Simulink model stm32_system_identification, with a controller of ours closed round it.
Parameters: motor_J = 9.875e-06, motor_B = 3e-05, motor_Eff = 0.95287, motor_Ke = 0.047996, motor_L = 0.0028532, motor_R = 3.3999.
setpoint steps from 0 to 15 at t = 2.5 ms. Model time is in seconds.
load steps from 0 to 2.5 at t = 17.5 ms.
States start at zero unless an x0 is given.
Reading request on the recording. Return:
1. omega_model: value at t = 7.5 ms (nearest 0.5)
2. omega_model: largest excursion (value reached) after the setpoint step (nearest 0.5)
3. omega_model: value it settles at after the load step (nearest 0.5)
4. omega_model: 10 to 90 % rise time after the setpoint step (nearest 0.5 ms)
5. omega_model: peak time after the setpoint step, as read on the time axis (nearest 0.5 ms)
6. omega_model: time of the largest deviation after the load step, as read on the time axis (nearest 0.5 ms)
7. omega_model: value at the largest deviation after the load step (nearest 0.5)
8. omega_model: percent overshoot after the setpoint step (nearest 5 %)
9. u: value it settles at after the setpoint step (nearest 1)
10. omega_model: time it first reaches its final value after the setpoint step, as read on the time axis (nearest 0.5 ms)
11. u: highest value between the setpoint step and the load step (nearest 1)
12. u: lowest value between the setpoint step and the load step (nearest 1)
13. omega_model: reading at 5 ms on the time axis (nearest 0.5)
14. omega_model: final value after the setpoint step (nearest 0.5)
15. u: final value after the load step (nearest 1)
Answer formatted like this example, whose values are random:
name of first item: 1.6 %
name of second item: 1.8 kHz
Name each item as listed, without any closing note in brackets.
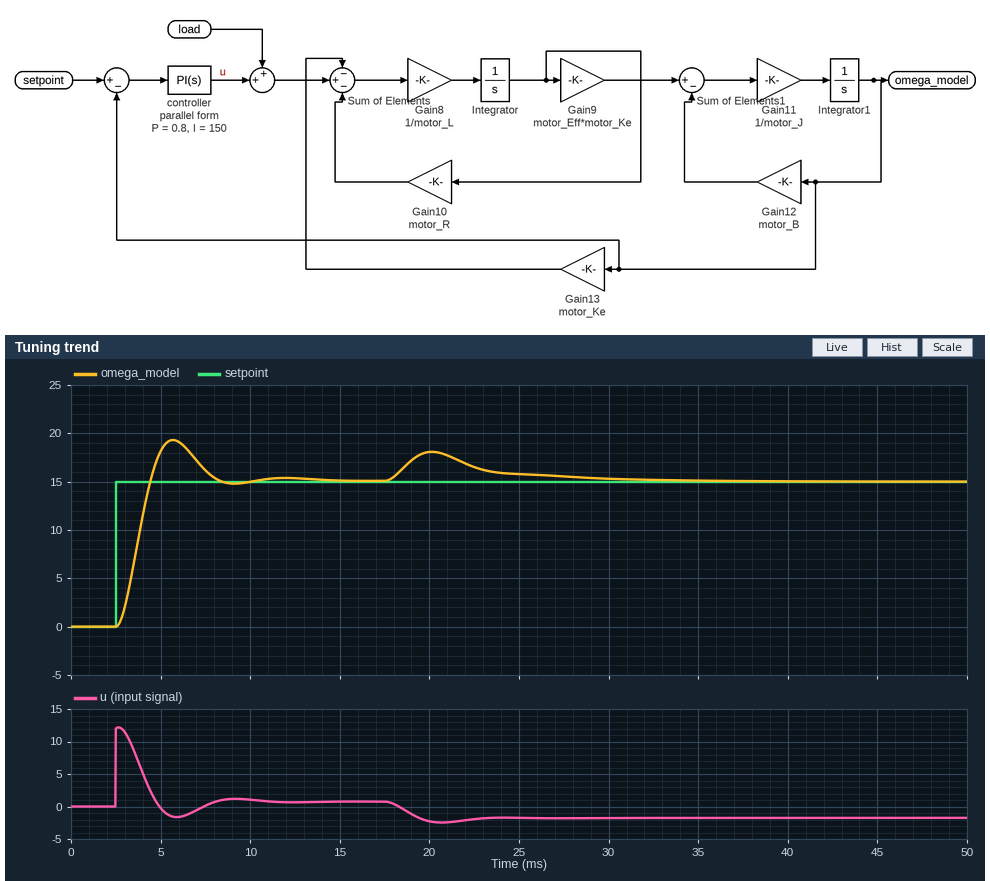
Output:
omega_model: value at t = 7.5 ms: 16.0
omega_model: largest excursion (value reached) after the setpoint step: 19.5
omega_model: value it settles at after the load step: 15.0
omega_model: 10 to 90 % rise time after the setpoint step: 1.5 ms
omega_model: peak time after the setpoint step, as read on the time axis: 5.5 ms
omega_model: time of the largest deviation after the load step, as read on the time axis: 20.0 ms
omega_model: value at the largest deviation after the load step: 18.0
omega_model: percent overshoot after the setpoint step: 30 %
u: value it settles at after the setpoint step: 1
omega_model: time it first reaches its final value after the setpoint step, as read on the time axis: 4.5 ms
u: highest value between the setpoint step and the load step: 12
u: lowest value between the setpoint step and the load step: -2
omega_model: reading at 5 ms on the time axis: 18.0
omega_model: final value after the setpoint step: 15.0
u: final value after the load step: -2
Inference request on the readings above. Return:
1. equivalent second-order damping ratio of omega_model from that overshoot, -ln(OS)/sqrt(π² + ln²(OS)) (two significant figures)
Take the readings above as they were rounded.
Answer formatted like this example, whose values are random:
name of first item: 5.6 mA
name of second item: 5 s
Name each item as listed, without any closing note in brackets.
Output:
equivalent second-order damping ratio of omega_model from that overshoot, -ln(OS)/sqrt(π² + ln²(OS)): 0.36
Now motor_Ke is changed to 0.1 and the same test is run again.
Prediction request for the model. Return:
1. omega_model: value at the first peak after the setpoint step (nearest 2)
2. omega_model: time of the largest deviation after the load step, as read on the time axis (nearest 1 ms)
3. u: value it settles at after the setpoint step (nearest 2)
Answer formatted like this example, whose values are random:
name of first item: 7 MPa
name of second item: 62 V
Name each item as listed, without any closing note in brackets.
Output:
omega_model: value at the first peak after the setpoint step: 20
omega_model: time of the largest deviation after the load step, as read on the time axis: 19 ms
u: value it settles at after the setpoint step: 2
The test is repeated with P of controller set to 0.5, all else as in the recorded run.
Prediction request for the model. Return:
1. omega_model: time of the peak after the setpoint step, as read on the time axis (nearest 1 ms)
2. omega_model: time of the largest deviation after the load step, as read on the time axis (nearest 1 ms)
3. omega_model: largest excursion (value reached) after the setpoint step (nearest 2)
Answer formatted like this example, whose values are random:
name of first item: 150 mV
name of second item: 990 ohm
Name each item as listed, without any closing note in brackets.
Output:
omega_model: time of the peak after the setpoint step, as read on the time axis: 7 ms
omega_model: time of the largest deviation after the load step, as read on the time axis: 21 ms
omega_model: largest excursion (value reached) after the setpoint step: 20
